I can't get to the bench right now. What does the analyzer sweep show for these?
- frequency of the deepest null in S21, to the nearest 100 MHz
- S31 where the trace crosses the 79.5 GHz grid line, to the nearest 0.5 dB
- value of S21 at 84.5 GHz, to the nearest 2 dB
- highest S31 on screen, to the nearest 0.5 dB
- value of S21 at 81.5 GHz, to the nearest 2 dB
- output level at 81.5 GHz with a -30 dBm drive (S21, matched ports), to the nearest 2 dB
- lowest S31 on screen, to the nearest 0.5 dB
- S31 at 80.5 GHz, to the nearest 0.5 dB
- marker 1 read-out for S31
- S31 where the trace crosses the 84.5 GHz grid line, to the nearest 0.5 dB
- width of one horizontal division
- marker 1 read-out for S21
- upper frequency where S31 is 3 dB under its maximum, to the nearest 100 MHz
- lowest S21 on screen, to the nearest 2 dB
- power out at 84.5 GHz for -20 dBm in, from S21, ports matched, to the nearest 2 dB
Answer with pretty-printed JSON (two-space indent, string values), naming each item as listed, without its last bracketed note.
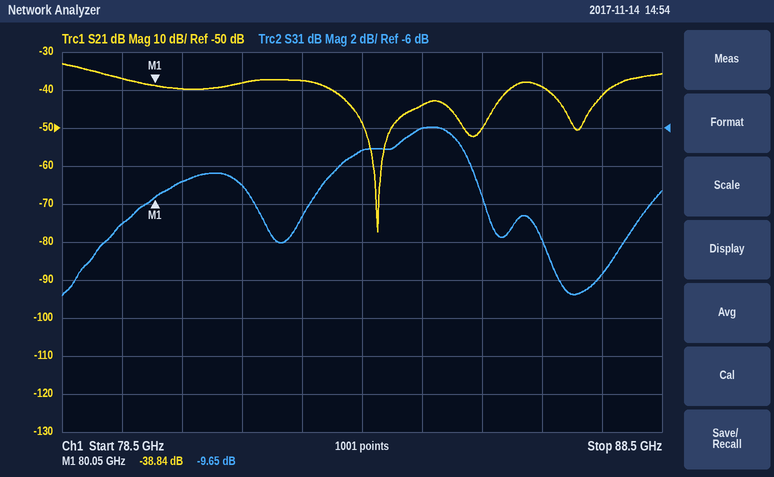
{
  "frequency of the deepest null in S21, to the nearest 100 MHz": "83.8 GHz",
  "S31 where the trace crosses the 79.5 GHz grid line, to the nearest 0.5 dB": "-11.0 dB",
  "value of S21 at 84.5 GHz, to the nearest 2 dB": "-44 dB",
  "highest S31 on screen, to the nearest 0.5 dB": "-6.0 dB",
  "value of S21 at 81.5 GHz, to the nearest 2 dB": "-38 dB",
  "output level at 81.5 GHz with a -30 dBm drive (S21, matched ports), to the nearest 2 dB": "-68 dBm",
  "lowest S31 on screen, to the nearest 0.5 dB": "-15.0 dB",
  "S31 at 80.5 GHz, to the nearest 0.5 dB": "-9.0 dB",
  "marker 1 read-out for S31": "-9.65 dB",
  "S31 where the trace crosses the 84.5 GHz grid line, to the nearest 0.5 dB": "-6.0 dB",
  "width of one horizontal division": "1 GHz",
  "marker 1 read-out for S21": "-38.84 dB",
  "upper frequency where S31 is 3 dB under its maximum, to the nearest 100 MHz": "85.4 GHz",
  "lowest S21 on screen, to the nearest 2 dB": "-78 dB",
  "power out at 84.5 GHz for -20 dBm in, from S21, ports matched, to the nearest 2 dB": "-64 dBm"
}
